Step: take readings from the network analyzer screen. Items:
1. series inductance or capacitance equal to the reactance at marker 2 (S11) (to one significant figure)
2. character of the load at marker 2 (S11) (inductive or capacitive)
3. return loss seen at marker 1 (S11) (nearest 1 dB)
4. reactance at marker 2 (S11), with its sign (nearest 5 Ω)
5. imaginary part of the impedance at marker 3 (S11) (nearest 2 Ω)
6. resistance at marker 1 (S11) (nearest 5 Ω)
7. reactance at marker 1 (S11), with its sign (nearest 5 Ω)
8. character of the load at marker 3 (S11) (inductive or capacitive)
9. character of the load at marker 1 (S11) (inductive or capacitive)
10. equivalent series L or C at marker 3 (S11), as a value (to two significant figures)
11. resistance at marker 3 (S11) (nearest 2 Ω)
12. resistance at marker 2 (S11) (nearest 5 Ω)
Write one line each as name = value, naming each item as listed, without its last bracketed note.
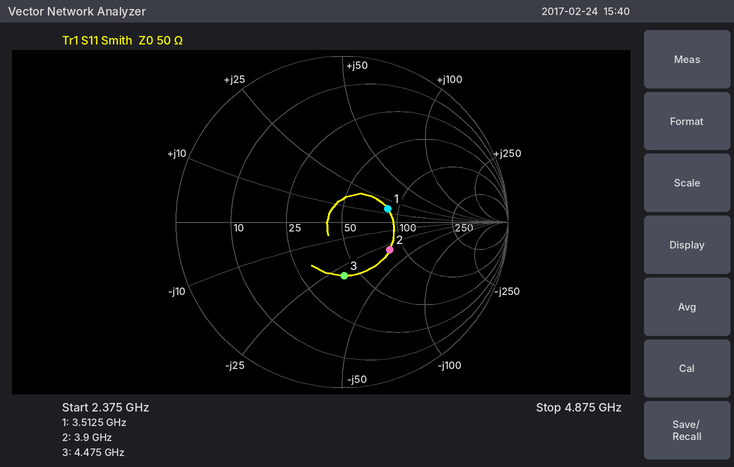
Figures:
series inductance or capacitance equal to the reactance at marker 2 (S11) = 1 pF
character of the load at marker 2 (S11) = capacitive
return loss seen at marker 1 (S11) = 11 dB
reactance at marker 2 (S11), with its sign = -30 Ω
imaginary part of the impedance at marker 3 (S11) = -30 Ω
resistance at marker 1 (S11) = 85 Ω
reactance at marker 1 (S11), with its sign = +15 Ω
character of the load at marker 3 (S11) = capacitive
character of the load at marker 1 (S11) = inductive
equivalent series L or C at marker 3 (S11), as a value = 1.2 pF
resistance at marker 3 (S11) = 42 Ω
resistance at marker 2 (S11) = 85 Ω
